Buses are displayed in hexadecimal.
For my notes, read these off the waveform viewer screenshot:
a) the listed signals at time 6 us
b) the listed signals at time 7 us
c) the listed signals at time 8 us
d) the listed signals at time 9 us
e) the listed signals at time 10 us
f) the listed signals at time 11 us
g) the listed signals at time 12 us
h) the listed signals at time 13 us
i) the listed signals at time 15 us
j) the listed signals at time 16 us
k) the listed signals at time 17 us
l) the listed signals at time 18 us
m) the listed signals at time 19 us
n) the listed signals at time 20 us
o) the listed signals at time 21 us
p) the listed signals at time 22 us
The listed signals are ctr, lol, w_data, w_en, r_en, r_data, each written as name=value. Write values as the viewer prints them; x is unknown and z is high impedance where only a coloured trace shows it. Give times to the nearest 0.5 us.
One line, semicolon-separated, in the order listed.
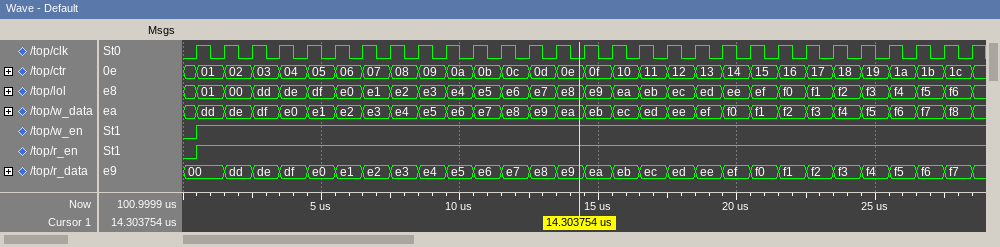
ctr=06, lol=e0, w_data=e2, w_en=1, r_en=1, r_data=e1; ctr=07, lol=e1, w_data=e3, w_en=1, r_en=1, r_data=e2; ctr=08, lol=e2, w_data=e4, w_en=1, r_en=1, r_data=e3; ctr=09, lol=e3, w_data=e5, w_en=1, r_en=1, r_data=e4; ctr=0a, lol=e4, w_data=e6, w_en=1, r_en=1, r_data=e5; ctr=0b, lol=e5, w_data=e7, w_en=1, r_en=1, r_data=e6; ctr=0c, lol=e6, w_data=e8, w_en=1, r_en=1, r_data=e7; ctr=0d, lol=e7, w_data=e9, w_en=1, r_en=1, r_data=e8; ctr=0f, lol=e9, w_data=eb, w_en=1, r_en=1, r_data=ea; ctr=10, lol=ea, w_data=ec, w_en=1, r_en=1, r_data=eb; ctr=11, lol=eb, w_data=ed, w_en=1, r_en=1, r_data=ec; ctr=12, lol=ec, w_data=ee, w_en=1, r_en=1, r_data=ed; ctr=13, lol=ed, w_data=ef, w_en=1, r_en=1, r_data=ee; ctr=14, lol=ee, w_data=f0, w_en=1, r_en=1, r_data=ef; ctr=15, lol=ef, w_data=f1, w_en=1, r_en=1, r_data=f0; ctr=16, lol=f0, w_data=f2, w_en=1, r_en=1, r_data=f1
